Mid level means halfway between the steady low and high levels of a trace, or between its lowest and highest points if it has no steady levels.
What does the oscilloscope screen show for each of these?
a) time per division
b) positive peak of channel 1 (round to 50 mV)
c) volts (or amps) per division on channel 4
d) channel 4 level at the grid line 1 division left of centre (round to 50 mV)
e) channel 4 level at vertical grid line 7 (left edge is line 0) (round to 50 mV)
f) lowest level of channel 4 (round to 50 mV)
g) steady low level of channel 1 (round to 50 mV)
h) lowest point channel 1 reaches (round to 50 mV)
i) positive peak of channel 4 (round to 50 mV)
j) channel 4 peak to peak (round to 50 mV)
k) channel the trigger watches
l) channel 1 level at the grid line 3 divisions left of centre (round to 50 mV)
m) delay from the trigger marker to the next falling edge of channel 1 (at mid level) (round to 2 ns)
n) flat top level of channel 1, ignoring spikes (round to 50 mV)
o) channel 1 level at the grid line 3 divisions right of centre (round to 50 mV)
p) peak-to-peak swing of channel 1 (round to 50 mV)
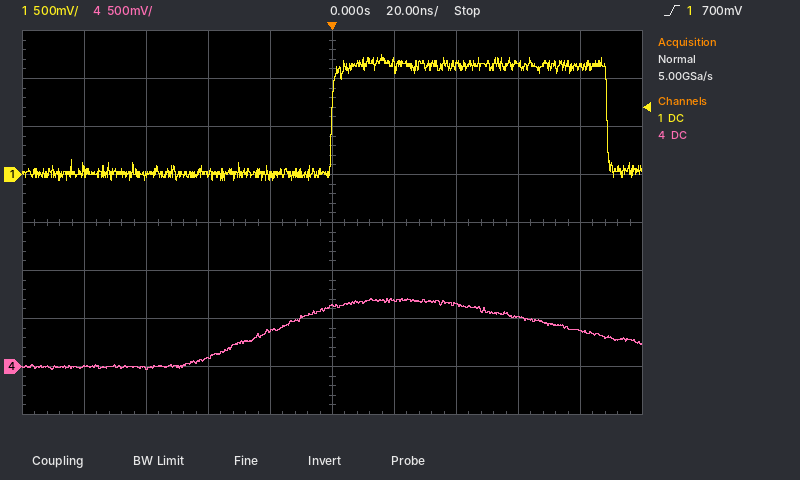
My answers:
20 ns
1.25 V
500 mV
350 mV
650 mV
-50 mV
0 mV
-50 mV
700 mV
750 mV
channel 1
0 mV
88 ns
1.15 V
1.15 V
1.30 V
